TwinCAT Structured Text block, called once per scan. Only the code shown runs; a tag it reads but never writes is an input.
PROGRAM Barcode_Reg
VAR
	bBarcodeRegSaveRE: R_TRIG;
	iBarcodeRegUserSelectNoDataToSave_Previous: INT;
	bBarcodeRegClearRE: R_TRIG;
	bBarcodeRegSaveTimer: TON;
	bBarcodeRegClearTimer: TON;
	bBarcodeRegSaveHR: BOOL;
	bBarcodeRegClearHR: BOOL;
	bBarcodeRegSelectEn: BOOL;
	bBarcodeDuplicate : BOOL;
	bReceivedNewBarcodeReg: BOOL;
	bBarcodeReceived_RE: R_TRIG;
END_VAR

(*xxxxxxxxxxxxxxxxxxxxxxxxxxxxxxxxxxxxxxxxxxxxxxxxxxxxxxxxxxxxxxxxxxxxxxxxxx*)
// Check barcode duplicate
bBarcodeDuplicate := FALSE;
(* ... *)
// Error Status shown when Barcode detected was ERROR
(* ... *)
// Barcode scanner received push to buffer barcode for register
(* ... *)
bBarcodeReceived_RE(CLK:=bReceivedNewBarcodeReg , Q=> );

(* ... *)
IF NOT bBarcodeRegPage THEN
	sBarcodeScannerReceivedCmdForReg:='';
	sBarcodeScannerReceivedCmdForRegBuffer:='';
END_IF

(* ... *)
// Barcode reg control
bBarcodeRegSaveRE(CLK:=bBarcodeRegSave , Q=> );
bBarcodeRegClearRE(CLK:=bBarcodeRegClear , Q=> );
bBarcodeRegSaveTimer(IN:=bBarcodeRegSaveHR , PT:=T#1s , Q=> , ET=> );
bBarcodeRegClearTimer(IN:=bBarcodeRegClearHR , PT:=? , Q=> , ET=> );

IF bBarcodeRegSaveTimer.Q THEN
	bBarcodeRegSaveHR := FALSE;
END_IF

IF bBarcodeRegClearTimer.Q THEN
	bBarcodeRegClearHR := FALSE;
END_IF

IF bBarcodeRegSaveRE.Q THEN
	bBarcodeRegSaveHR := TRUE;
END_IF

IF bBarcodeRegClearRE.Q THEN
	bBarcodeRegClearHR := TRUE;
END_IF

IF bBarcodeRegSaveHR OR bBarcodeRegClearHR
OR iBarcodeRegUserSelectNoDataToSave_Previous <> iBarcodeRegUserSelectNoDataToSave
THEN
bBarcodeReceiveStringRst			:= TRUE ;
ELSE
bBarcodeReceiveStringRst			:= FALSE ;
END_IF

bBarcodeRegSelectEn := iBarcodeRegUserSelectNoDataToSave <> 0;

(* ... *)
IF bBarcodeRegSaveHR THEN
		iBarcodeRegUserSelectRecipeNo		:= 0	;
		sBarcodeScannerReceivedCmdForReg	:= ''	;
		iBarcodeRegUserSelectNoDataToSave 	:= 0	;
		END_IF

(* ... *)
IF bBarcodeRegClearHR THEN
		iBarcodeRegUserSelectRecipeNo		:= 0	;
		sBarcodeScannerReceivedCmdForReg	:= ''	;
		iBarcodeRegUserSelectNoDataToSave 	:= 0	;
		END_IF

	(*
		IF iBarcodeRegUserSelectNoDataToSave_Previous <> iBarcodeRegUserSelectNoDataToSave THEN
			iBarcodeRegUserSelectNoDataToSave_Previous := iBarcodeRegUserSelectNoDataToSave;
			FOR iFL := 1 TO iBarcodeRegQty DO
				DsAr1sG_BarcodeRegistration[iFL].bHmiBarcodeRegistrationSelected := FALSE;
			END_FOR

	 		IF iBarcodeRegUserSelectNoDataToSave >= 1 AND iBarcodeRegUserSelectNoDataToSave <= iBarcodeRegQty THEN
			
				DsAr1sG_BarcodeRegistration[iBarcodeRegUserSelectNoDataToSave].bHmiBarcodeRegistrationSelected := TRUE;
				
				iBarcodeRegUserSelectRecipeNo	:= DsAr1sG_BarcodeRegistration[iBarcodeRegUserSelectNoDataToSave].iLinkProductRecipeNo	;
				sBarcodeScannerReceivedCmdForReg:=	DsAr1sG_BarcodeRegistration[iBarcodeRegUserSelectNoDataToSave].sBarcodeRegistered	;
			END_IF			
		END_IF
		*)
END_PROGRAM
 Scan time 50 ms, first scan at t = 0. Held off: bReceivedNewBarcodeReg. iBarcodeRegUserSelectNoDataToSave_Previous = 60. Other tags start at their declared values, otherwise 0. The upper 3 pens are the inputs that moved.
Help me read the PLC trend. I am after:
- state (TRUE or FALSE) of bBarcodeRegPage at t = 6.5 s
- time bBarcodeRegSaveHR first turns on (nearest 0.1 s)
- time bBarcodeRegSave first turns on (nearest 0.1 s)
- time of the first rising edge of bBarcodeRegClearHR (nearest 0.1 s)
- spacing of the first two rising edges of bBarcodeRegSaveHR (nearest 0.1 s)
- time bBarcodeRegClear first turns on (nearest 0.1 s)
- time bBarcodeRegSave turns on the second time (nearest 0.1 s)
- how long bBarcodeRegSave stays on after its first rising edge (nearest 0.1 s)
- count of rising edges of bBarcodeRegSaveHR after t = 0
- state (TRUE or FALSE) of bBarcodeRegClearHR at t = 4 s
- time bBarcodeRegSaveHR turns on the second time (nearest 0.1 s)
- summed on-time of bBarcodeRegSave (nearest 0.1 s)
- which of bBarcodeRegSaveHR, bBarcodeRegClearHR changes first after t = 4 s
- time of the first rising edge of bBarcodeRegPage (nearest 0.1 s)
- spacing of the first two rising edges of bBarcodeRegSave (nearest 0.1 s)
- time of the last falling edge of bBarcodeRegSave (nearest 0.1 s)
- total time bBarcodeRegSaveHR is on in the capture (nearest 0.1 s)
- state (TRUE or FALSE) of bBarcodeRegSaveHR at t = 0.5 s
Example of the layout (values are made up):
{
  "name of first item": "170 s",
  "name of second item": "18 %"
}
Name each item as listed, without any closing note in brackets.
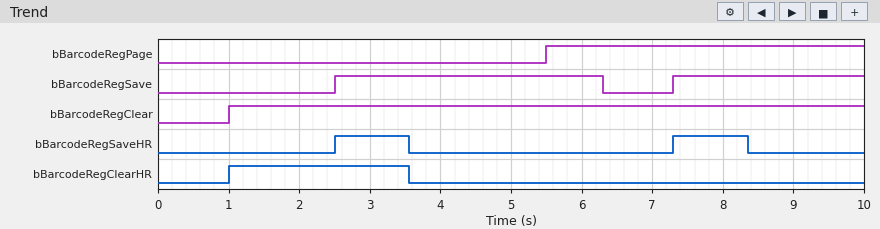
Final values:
{
  "state (TRUE or FALSE) of bBarcodeRegPage at t = 6.5 s": "TRUE",
  "time bBarcodeRegSaveHR first turns on": "2.5 s",
  "time bBarcodeRegSave first turns on": "2.5 s",
  "time of the first rising edge of bBarcodeRegClearHR": "1.0 s",
  "spacing of the first two rising edges of bBarcodeRegSaveHR": "4.8 s",
  "time bBarcodeRegClear first turns on": "1.0 s",
  "time bBarcodeRegSave turns on the second time": "7.3 s",
  "how long bBarcodeRegSave stays on after its first rising edge": "3.8 s",
  "count of rising edges of bBarcodeRegSaveHR after t = 0": "2",
  "state (TRUE or FALSE) of bBarcodeRegClearHR at t = 4 s": "FALSE",
  "time bBarcodeRegSaveHR turns on the second time": "7.3 s",
  "summed on-time of bBarcodeRegSave": "6.5 s",
  "which of bBarcodeRegSaveHR, bBarcodeRegClearHR changes first after t = 4 s": "bBarcodeRegSaveHR",
  "time of the first rising edge of bBarcodeRegPage": "5.5 s",
  "spacing of the first two rising edges of bBarcodeRegSave": "4.8 s",
  "time of the last falling edge of bBarcodeRegSave": "6.3 s",
  "total time bBarcodeRegSaveHR is on in the capture": "2.1 s",
  "state (TRUE or FALSE) of bBarcodeRegSaveHR at t = 0.5 s": "FALSE"
}
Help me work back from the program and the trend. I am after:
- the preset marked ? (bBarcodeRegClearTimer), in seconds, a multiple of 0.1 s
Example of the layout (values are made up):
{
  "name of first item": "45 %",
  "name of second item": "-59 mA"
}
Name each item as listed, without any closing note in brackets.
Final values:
{
  "the preset marked ? (bBarcodeRegClearTimer), in seconds, a multiple of 0.1 s": "2.5 s"
}
